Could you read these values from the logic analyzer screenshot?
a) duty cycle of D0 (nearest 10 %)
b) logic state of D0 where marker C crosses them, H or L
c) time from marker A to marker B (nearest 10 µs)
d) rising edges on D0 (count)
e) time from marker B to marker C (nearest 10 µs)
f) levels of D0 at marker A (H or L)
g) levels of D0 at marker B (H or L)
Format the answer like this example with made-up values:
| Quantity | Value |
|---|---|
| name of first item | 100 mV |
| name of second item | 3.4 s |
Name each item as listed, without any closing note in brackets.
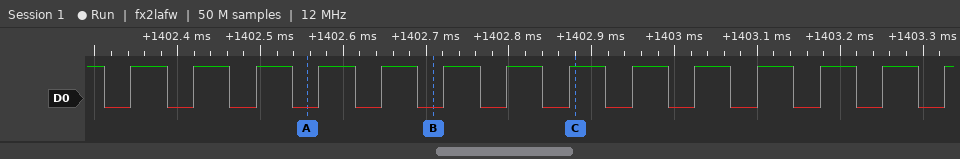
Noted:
| Quantity | Value |
|---|---|
| duty cycle of D0 | 60 % |
| logic state of D0 where marker C crosses them, H or L | D0=H |
| time from marker A to marker B | 150 µs |
| rising edges on D0 | 14 |
| time from marker B to marker C | 170 µs |
| levels of D0 at marker A | D0=L |
| levels of D0 at marker B | D0=L |
